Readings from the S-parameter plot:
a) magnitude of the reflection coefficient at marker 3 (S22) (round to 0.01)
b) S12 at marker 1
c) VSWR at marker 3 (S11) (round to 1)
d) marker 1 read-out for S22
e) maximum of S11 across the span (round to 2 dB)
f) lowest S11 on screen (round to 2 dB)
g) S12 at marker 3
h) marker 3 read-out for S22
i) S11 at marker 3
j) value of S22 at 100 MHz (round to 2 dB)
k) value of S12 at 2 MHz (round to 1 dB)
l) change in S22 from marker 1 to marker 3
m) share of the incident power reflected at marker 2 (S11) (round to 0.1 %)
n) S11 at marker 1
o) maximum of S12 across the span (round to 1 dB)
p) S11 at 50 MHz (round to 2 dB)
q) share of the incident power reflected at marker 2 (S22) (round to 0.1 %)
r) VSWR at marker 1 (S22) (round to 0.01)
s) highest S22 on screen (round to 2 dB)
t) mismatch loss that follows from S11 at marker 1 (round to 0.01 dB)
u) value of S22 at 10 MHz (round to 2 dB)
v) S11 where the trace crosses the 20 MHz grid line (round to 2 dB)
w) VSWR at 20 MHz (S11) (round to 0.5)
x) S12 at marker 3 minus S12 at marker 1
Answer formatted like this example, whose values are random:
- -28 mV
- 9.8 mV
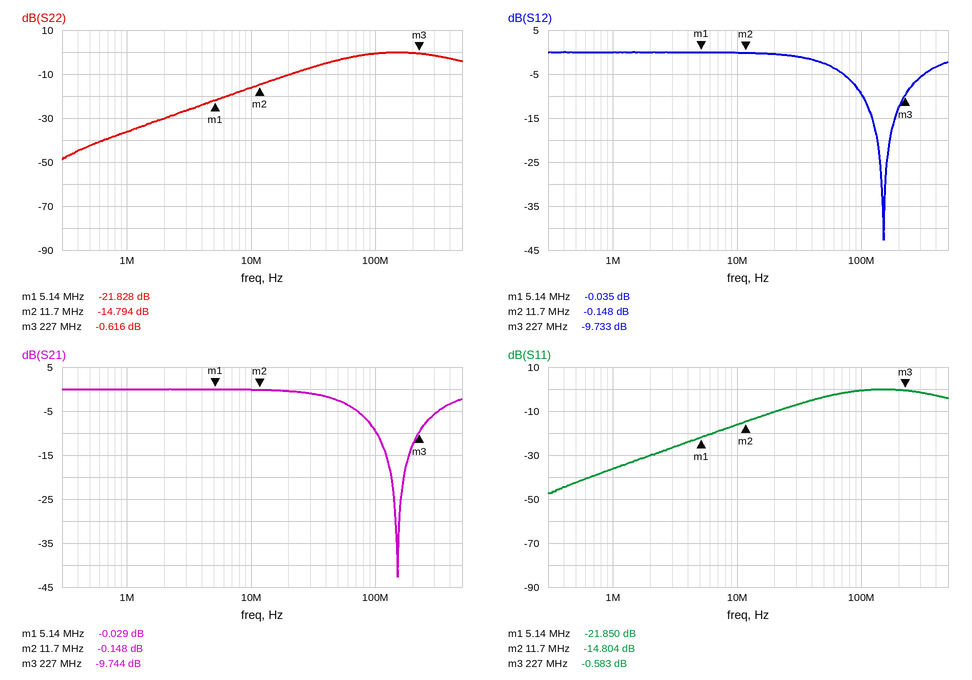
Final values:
- 0.93
- -0.035 dB
- 30
- -21.828 dB
- 0 dB
- -48 dB
- -9.733 dB
- -0.616 dB
- -0.583 dB
- 0 dB
- 0 dB
- 21.212 dB
- 3.3 %
- -21.850 dB
- 0 dB
- -4 dB
- 3.3 %
- 1.18
- 0 dB
- 0.03 dB
- -16 dB
- -10 dB
- 2.0
- -9.698 dB
